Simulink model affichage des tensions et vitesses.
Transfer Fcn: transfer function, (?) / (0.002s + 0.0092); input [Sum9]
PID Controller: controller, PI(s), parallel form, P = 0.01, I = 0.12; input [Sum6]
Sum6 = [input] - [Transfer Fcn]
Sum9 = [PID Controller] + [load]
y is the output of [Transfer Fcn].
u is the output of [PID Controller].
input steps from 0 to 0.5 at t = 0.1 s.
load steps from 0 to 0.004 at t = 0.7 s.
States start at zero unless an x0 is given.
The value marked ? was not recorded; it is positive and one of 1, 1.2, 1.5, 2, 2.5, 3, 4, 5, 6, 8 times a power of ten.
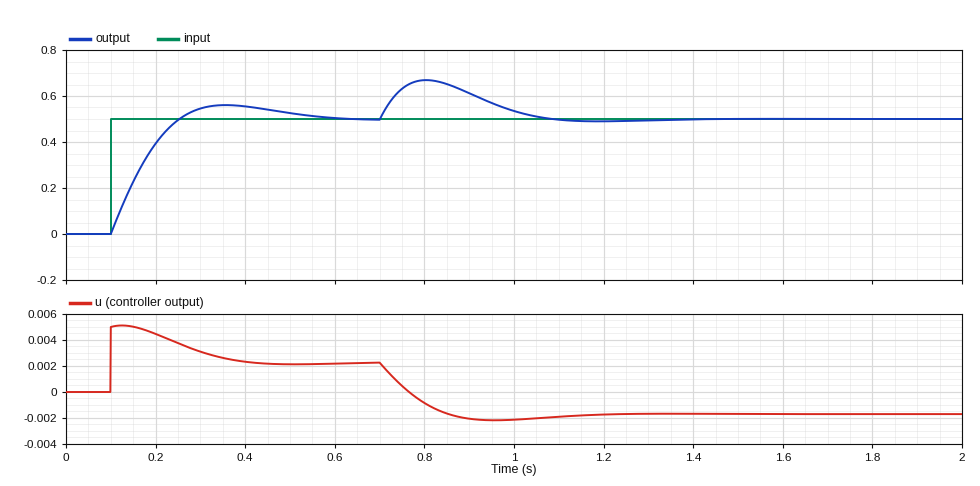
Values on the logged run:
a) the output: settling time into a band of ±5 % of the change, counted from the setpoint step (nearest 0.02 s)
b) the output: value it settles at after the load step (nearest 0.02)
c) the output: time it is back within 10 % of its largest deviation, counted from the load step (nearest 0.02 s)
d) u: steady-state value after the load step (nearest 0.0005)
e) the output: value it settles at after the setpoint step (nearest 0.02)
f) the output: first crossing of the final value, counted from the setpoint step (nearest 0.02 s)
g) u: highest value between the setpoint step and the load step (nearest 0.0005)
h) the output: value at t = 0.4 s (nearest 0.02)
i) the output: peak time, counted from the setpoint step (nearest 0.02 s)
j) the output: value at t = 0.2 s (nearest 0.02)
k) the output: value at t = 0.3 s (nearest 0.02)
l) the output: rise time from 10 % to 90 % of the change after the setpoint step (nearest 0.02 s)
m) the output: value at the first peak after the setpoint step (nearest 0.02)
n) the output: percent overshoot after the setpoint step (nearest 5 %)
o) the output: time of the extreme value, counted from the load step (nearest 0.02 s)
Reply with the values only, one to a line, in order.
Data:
0.40 s
0.50
0.34 s
-0.0015
0.50
0.16 s
0.0050
0.56
0.26 s
0.40
0.54
0.12 s
0.56
10 %
0.10 s
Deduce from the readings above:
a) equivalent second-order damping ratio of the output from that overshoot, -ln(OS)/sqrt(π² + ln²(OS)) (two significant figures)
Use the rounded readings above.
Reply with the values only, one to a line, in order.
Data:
0.59
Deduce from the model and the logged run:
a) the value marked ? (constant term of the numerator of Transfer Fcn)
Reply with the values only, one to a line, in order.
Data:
2
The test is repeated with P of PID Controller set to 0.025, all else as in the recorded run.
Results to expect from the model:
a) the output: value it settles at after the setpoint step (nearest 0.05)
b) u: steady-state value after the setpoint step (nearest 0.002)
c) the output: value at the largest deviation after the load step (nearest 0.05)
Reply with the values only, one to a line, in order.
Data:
0.50
0.002
0.60
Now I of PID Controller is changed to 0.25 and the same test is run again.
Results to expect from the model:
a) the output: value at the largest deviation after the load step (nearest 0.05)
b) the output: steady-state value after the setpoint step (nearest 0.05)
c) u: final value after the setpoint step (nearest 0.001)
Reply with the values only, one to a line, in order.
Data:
0.65
0.50
0.002
